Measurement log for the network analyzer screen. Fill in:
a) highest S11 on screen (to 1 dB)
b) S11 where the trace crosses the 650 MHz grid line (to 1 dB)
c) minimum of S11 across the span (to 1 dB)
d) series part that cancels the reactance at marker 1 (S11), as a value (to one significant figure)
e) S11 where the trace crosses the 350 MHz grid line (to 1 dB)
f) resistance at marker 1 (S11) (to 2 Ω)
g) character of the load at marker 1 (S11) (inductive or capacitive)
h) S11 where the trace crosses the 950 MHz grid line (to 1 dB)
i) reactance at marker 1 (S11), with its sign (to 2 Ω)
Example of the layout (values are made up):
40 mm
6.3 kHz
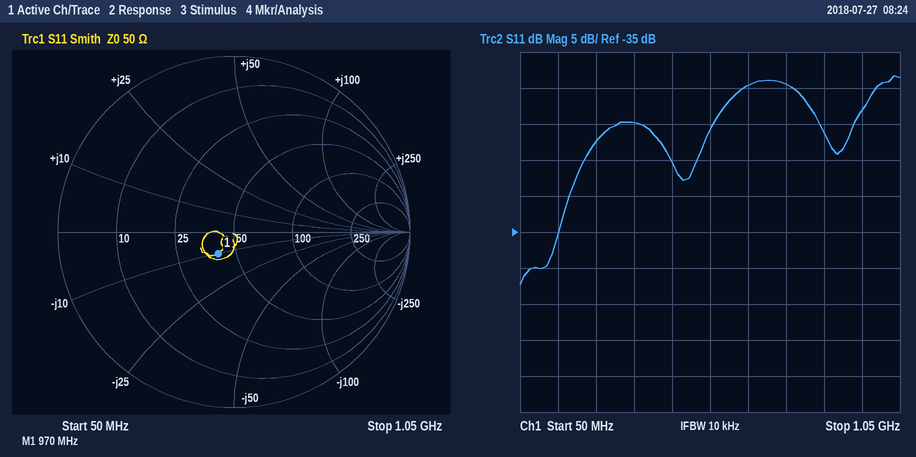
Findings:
-13 dB
-15 dB
-42 dB
2 nH
-20 dB
40 Ω
capacitive
-18 dB
-10 Ω
